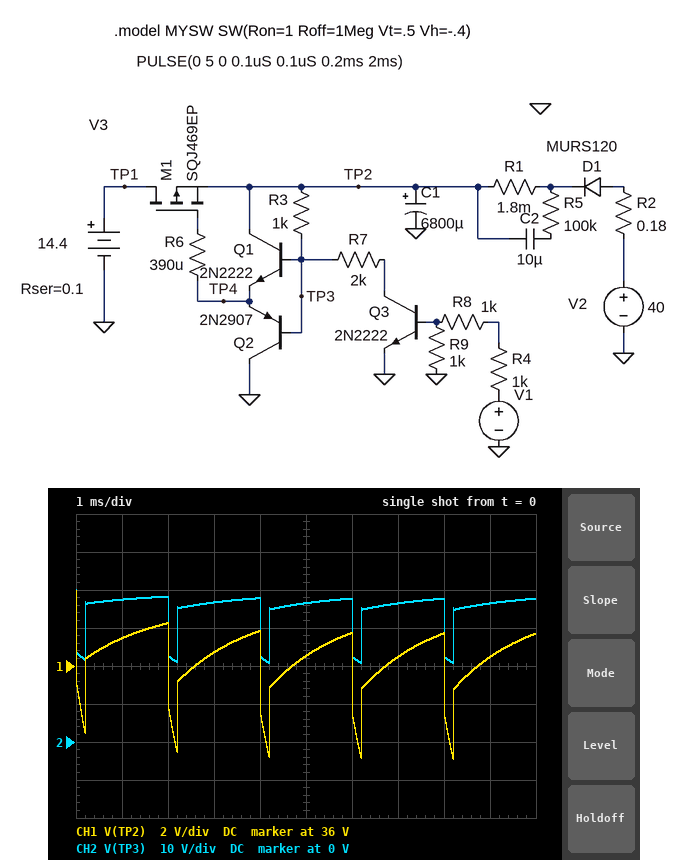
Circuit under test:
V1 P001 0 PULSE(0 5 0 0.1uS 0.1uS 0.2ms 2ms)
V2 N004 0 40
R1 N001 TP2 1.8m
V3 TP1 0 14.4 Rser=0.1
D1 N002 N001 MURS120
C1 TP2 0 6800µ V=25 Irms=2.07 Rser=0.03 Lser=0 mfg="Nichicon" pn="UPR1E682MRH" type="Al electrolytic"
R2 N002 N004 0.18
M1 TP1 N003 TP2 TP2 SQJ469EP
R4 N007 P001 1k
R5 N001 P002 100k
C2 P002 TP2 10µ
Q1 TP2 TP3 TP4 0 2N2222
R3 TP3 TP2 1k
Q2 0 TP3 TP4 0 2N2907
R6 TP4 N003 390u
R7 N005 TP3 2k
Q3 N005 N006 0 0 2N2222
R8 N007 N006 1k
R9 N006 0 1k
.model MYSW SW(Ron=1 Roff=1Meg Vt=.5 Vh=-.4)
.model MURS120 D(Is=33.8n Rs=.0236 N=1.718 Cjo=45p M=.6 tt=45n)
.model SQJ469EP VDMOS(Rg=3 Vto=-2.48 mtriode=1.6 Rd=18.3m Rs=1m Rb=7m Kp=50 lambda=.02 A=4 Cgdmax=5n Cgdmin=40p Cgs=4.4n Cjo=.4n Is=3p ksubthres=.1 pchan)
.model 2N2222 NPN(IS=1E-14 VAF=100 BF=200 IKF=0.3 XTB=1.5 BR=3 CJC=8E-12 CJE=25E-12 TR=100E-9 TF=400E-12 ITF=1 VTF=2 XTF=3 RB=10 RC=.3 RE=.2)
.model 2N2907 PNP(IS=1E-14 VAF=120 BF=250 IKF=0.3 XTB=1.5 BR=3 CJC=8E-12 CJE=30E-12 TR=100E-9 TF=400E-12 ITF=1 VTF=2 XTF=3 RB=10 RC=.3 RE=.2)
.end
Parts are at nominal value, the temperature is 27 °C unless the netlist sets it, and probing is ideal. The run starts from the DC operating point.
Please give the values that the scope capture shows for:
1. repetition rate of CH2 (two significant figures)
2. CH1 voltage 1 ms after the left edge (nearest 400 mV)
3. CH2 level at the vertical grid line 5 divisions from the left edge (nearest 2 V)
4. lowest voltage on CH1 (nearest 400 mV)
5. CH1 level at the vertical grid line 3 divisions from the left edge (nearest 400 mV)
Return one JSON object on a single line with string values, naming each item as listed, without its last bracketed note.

{"repetition rate of CH2": "500 Hz", "CH1 voltage 1 ms after the left edge": "37.6 V", "CH2 level at the vertical grid line 5 divisions from the left edge": "36 V", "lowest voltage on CH1": "31.2 V", "CH1 level at the vertical grid line 3 divisions from the left edge": "36.8 V"}
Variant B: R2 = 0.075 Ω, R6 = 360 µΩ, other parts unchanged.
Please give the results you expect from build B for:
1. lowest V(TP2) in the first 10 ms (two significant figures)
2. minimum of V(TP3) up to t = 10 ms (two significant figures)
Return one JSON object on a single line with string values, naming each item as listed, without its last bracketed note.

{"lowest V(TP2) in the first 10 ms": "33 V", "minimum of V(TP3) up to t = 10 ms": "22 V"}
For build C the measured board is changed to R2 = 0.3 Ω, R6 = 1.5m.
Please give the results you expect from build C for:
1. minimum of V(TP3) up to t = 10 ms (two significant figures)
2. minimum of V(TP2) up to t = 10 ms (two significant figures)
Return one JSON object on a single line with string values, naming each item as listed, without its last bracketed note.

{"minimum of V(TP3) up to t = 10 ms": "20 V", "minimum of V(TP2) up to t = 10 ms": "30 V"}
